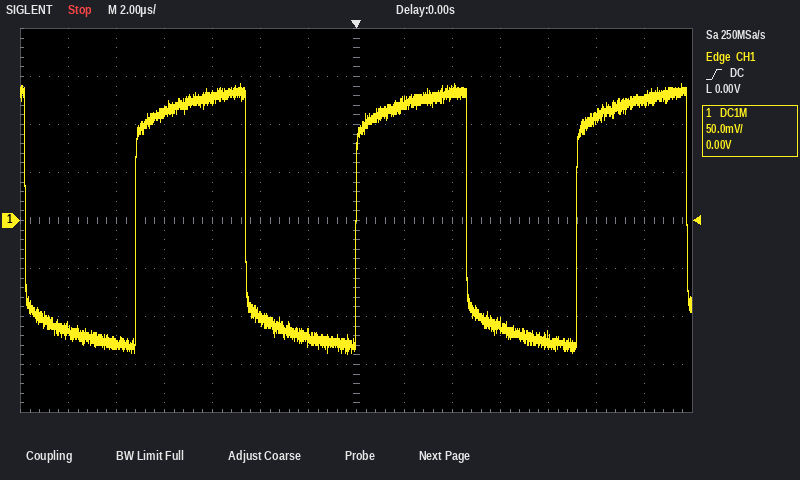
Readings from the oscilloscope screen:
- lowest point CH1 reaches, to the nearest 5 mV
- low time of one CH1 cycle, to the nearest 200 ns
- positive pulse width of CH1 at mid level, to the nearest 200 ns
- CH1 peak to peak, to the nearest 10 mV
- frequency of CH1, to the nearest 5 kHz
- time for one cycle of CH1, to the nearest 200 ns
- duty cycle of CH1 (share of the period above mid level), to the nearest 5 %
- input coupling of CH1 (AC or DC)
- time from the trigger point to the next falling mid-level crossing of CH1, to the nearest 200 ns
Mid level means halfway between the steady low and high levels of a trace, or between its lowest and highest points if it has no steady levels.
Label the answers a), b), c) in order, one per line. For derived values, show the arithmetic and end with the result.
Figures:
a) -140 mV
b) 4.6 µs
c) 4.6 µs
d) 280 mV
e) 1 / 9.2 µs ≈ 109 kHz, so 110 kHz to the nearest 5 kHz
f) 9.2 µs
g) 4.6 µs / 9.2 µs ≈ 50 %
h) DC
i) 4.6 µs
